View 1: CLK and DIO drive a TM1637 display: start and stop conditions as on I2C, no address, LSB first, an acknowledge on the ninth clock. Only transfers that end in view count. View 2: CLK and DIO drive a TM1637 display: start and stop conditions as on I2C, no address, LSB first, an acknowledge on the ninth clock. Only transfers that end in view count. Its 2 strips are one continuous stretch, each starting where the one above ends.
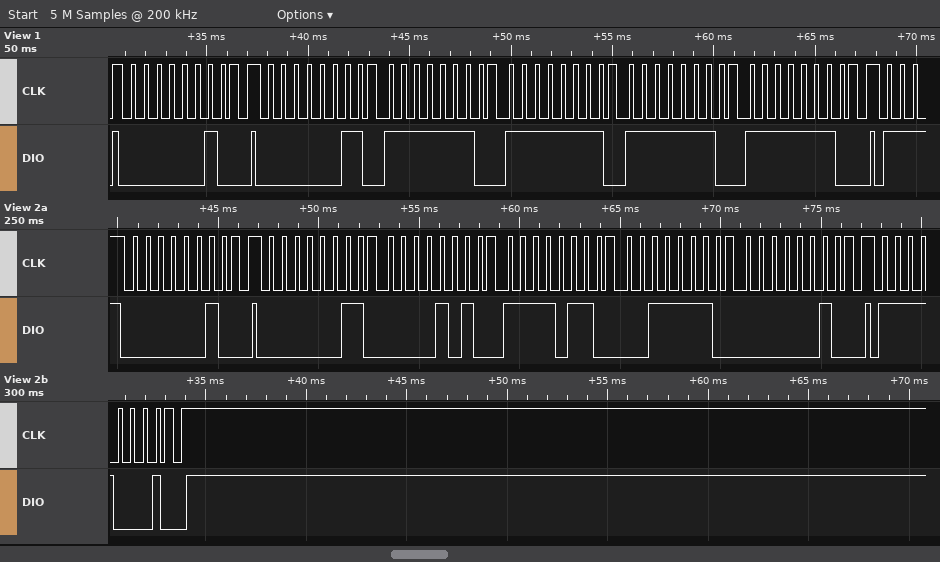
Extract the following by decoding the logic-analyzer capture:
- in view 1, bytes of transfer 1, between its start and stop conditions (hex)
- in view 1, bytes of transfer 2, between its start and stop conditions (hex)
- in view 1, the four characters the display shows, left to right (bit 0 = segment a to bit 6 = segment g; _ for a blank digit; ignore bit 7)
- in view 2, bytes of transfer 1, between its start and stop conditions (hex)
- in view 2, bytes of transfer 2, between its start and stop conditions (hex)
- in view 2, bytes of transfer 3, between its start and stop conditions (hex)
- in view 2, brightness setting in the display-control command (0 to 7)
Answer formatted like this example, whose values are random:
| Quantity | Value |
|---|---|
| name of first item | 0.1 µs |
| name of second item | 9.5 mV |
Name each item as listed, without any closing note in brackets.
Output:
| Quantity | Value |
|---|---|
| in view 1, bytes of transfer 1, between its start and stop conditions | 40 |
| in view 1, bytes of transfer 2, between its start and stop conditions | C0 7F FF 7F 7F |
| in view 1, the four characters the display shows, left to right | 8888 |
| in view 2, bytes of transfer 1, between its start and stop conditions | 40 |
| in view 2, bytes of transfer 2, between its start and stop conditions | C0 50 6F 7C 40 |
| in view 2, bytes of transfer 3, between its start and stop conditions | 8F |
| in view 2, brightness setting in the display-control command | 7 |
